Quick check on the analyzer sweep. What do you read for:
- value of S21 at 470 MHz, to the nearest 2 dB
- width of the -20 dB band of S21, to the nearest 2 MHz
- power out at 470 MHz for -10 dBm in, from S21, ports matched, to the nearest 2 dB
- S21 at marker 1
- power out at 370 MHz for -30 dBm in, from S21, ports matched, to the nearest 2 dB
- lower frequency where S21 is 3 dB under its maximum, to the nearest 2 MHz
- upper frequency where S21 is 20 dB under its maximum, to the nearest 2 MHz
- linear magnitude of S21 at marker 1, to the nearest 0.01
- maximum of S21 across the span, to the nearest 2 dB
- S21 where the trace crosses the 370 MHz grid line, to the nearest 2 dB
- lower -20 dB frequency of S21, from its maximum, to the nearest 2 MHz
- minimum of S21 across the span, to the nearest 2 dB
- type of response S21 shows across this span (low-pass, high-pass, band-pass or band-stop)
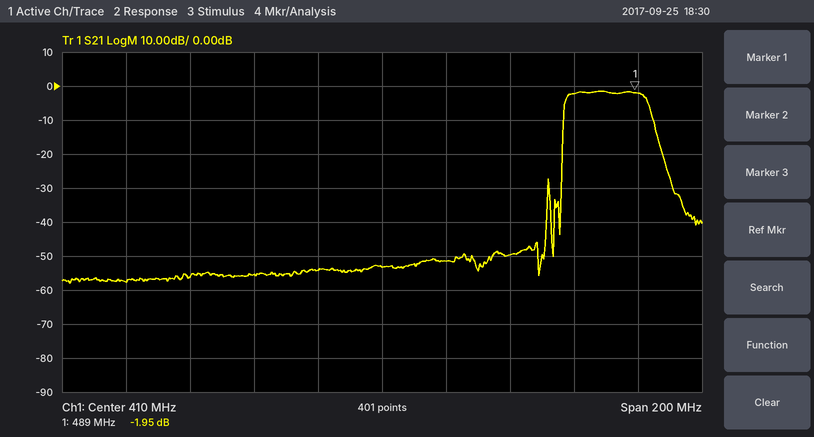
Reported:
-2 dB
32 MHz
-12 dBm
-1.95 dB
-86 dBm
468 MHz
498 MHz
0.80
-2 dB
-56 dB
466 MHz
-58 dB
band-pass
